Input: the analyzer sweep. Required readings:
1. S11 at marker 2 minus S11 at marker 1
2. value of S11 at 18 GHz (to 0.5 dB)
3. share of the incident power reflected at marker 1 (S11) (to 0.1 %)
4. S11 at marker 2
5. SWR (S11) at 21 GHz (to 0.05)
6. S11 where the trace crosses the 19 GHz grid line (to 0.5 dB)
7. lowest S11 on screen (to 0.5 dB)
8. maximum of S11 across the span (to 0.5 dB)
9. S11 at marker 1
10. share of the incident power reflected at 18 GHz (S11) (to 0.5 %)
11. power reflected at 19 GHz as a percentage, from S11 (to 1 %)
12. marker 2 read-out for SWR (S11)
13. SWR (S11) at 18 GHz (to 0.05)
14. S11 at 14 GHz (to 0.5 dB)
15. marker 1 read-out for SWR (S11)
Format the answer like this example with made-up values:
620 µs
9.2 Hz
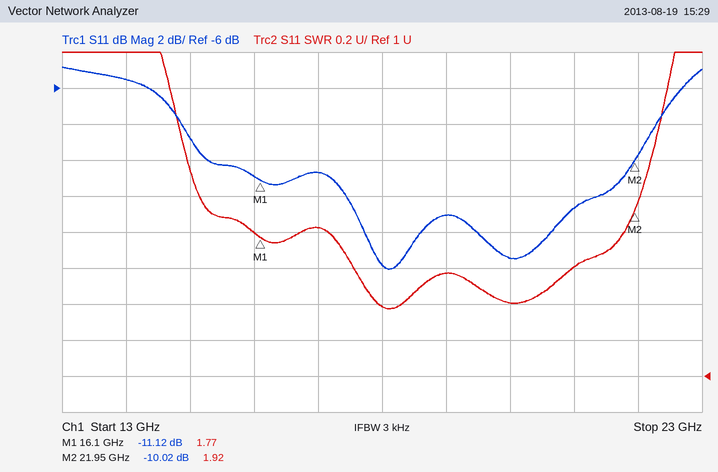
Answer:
1.10 dB
-16.0 dB
7.7 %
-10.02 dB
1.60
-13.0 dB
-16.0 dB
-5.0 dB
-11.12 dB
2.5 %
5 %
1.92
1.40
-5.5 dB
1.77
